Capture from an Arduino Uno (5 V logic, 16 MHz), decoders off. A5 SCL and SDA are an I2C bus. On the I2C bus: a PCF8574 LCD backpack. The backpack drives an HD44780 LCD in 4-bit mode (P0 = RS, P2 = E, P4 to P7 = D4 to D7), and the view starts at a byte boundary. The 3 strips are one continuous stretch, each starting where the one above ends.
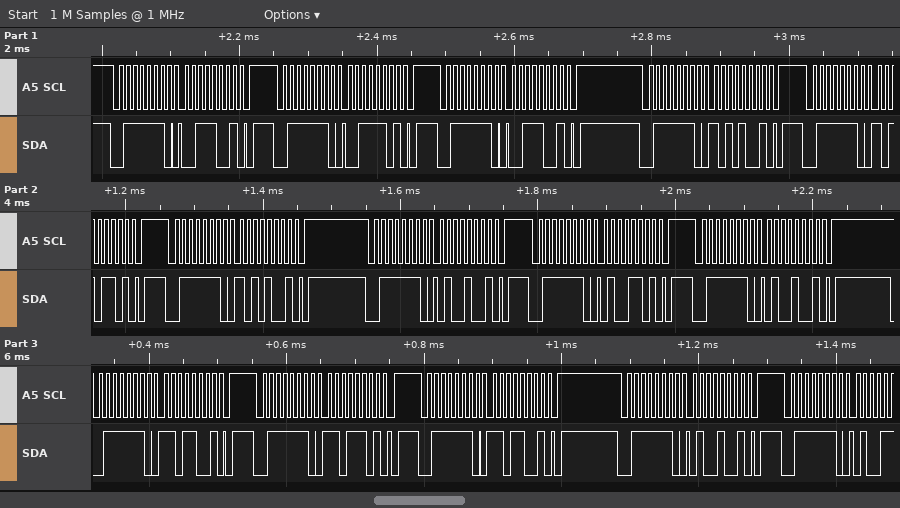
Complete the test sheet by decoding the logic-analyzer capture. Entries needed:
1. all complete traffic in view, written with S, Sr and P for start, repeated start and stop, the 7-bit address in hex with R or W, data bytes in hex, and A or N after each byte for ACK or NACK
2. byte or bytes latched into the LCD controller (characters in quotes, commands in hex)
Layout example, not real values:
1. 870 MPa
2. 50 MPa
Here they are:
1. S 3FW A 39 A P S 3FW A 3D A P S 3FW A 39 A P S 3FW A A9 A P S 3FW A AD A P S 3FW A A9 A P S 3FW A 49 A P S 3FW A 4D A P S 3FW A 49 A P S 3FW A D9 A P S 3FW A DD A P S 3FW A D9 A P S 3FW A 49 A P S 3FW A
2. ':' 'M'
